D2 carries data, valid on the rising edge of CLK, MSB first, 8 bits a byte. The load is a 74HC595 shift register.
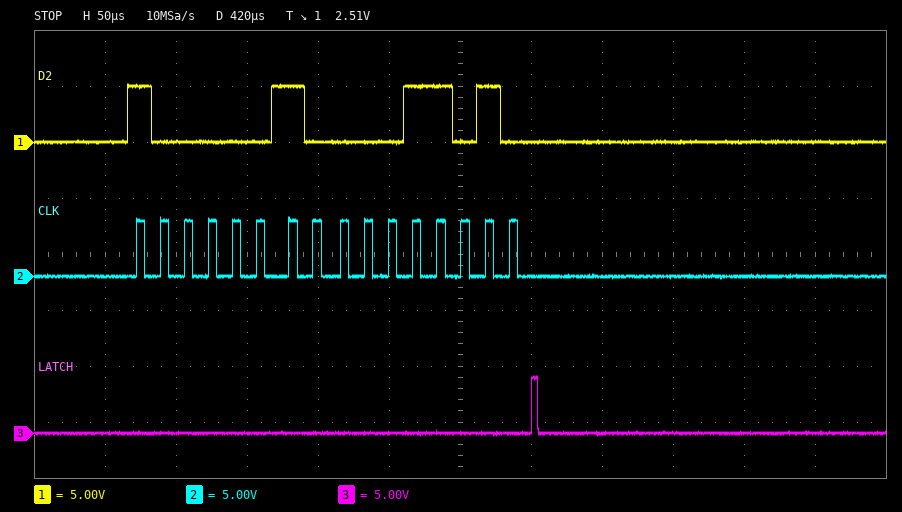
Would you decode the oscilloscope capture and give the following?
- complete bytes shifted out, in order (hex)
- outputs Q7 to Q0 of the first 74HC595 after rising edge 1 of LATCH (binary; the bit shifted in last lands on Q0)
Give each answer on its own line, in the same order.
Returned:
82 1A
00011010
